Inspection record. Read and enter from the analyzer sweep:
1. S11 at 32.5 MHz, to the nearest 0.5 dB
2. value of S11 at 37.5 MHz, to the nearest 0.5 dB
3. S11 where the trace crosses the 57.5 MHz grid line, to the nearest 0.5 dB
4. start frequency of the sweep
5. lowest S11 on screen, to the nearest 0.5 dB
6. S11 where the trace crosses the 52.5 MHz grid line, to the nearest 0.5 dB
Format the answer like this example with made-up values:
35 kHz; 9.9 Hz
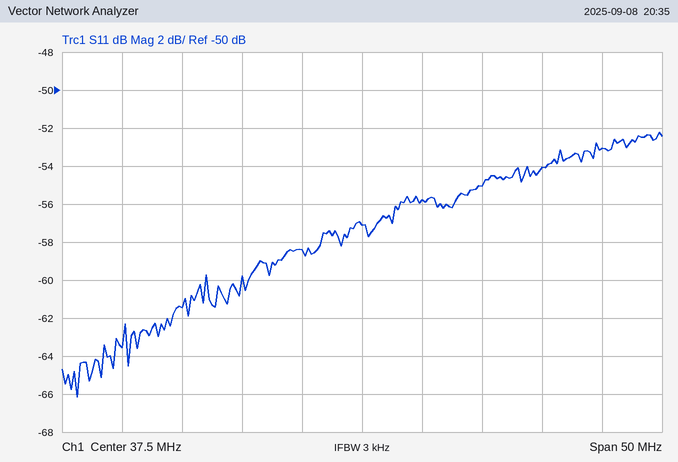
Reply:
-58.5 dB; -57.0 dB; -53.0 dB; 12.5 MHz; -66.0 dB; -54.0 dB
